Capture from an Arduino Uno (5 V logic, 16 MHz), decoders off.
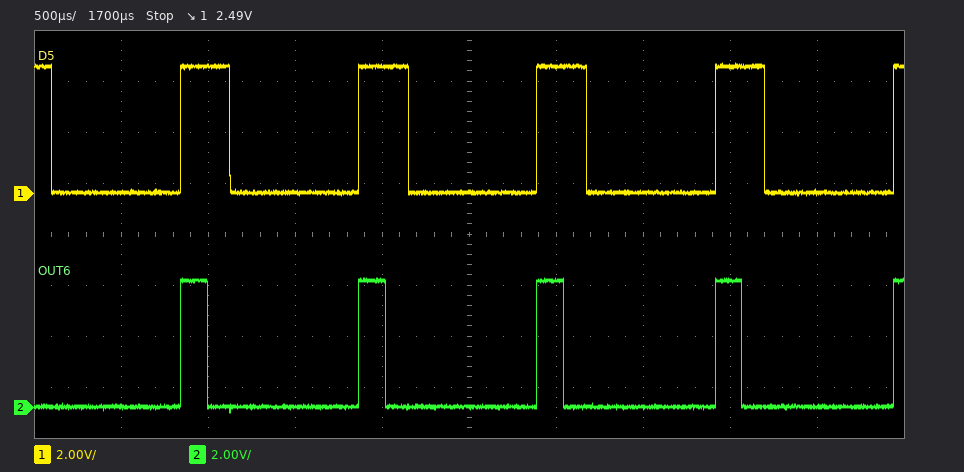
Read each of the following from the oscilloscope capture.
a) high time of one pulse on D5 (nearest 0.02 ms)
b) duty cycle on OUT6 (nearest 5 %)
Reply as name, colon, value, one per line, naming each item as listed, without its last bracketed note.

high time of one pulse on D5: 0.28 ms
duty cycle on OUT6: 15 %
